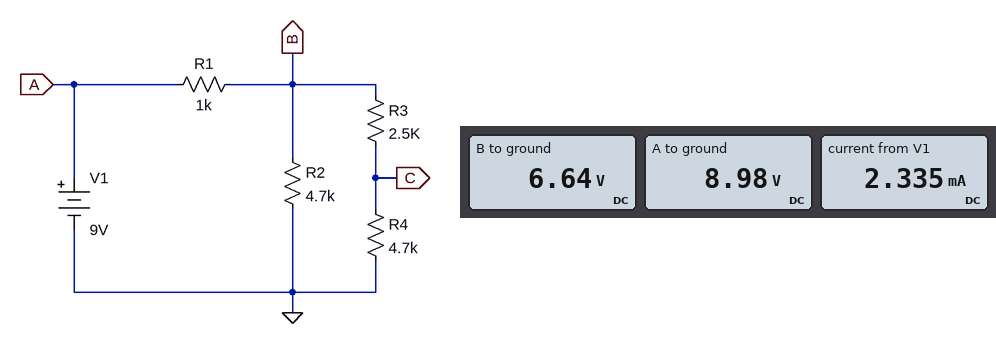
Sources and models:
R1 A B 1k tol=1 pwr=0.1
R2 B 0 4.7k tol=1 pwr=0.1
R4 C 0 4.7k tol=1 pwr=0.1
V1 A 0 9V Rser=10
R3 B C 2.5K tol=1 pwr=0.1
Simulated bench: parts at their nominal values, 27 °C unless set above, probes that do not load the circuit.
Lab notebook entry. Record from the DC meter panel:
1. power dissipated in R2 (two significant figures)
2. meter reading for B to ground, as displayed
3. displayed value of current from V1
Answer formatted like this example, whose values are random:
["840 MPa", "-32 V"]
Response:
["9.4 mW", "6.64 V", "2.335 mA"]
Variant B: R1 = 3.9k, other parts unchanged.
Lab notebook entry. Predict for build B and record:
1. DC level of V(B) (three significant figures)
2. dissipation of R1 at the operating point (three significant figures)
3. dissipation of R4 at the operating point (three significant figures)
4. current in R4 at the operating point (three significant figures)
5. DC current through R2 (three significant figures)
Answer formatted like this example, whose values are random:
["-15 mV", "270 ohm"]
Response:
["3.79 V", "6.93 mW", "1.30 mW", "526 µA", "806 µA"]
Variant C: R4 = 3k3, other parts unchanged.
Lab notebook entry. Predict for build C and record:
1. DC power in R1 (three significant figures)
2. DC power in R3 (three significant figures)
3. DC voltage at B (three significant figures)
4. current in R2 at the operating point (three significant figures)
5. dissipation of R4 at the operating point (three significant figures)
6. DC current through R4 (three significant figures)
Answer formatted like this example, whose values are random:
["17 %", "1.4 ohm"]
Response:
["6.23 mW", "3.12 mW", "6.48 V", "1.38 mA", "4.12 mW", "1.12 mA"]
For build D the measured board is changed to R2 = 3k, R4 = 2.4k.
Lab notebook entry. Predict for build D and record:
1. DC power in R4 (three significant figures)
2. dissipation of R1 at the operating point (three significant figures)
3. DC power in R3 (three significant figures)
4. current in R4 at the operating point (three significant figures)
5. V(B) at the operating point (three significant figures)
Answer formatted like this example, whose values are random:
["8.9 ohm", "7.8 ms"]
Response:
["3.40 mW", "9.83 mW", "3.54 mW", "1.19 mA", "5.83 V"]
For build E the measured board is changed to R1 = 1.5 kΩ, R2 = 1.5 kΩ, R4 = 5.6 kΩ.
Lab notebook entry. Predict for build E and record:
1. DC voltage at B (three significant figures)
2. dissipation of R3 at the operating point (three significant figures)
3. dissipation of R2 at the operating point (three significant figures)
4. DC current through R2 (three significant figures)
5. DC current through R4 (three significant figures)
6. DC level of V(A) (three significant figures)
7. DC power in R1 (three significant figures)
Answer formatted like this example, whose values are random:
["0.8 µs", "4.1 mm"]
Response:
["4.10 V", "642 µW", "11.2 mW", "2.74 mA", "507 µA", "8.97 V", "15.8 mW"]
